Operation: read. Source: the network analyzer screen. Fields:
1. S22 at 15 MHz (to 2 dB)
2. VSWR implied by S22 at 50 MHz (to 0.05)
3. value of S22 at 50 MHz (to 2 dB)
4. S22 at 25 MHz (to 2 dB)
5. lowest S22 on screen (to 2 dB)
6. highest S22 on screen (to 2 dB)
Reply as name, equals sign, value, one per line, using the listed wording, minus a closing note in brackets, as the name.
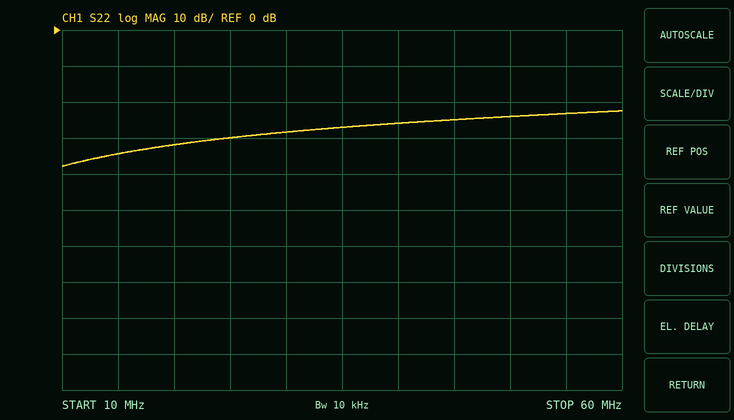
S22 at 15 MHz = -34 dB
VSWR implied by S22 at 50 MHz = 1.15
value of S22 at 50 MHz = -24 dB
S22 at 25 MHz = -30 dB
lowest S22 on screen = -38 dB
highest S22 on screen = -22 dB
